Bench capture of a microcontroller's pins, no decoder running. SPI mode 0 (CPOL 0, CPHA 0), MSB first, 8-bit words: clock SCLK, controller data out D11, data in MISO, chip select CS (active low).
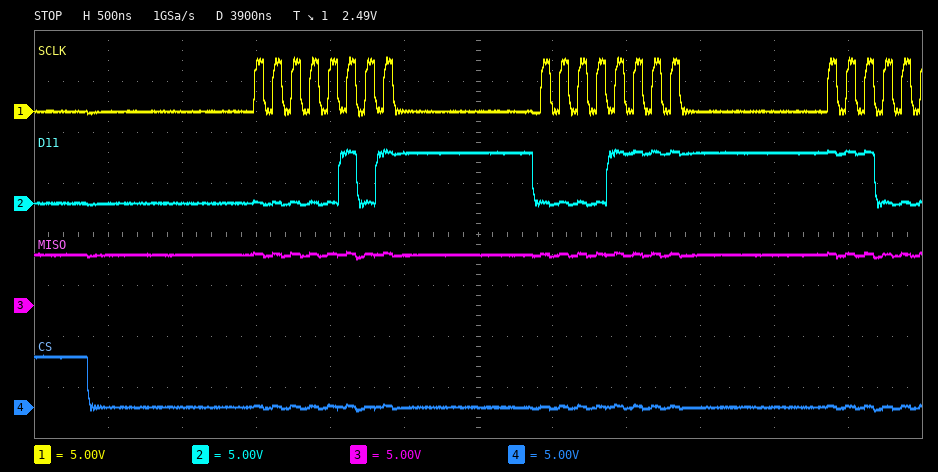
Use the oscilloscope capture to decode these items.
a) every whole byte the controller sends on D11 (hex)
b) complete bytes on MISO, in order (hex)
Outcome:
05 0F
FF FF
